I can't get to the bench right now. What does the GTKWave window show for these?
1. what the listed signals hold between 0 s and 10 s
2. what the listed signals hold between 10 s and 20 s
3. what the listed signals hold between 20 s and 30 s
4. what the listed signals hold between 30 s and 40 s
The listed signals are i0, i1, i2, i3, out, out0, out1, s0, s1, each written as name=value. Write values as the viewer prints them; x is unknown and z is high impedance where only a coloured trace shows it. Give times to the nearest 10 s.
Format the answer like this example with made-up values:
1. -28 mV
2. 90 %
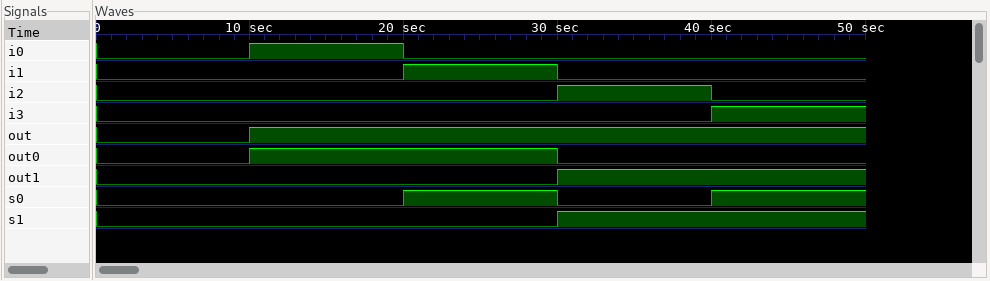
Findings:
1. i0=0, i1=0, i2=0, i3=0, out=0, out0=0, out1=0, s0=0, s1=0
2. i0=1, i1=0, i2=0, i3=0, out=1, out0=1, out1=0, s0=0, s1=0
3. i0=0, i1=1, i2=0, i3=0, out=1, out0=1, out1=0, s0=1, s1=0
4. i0=0, i1=0, i2=1, i3=0, out=1, out0=0, out1=1, s0=0, s1=1
